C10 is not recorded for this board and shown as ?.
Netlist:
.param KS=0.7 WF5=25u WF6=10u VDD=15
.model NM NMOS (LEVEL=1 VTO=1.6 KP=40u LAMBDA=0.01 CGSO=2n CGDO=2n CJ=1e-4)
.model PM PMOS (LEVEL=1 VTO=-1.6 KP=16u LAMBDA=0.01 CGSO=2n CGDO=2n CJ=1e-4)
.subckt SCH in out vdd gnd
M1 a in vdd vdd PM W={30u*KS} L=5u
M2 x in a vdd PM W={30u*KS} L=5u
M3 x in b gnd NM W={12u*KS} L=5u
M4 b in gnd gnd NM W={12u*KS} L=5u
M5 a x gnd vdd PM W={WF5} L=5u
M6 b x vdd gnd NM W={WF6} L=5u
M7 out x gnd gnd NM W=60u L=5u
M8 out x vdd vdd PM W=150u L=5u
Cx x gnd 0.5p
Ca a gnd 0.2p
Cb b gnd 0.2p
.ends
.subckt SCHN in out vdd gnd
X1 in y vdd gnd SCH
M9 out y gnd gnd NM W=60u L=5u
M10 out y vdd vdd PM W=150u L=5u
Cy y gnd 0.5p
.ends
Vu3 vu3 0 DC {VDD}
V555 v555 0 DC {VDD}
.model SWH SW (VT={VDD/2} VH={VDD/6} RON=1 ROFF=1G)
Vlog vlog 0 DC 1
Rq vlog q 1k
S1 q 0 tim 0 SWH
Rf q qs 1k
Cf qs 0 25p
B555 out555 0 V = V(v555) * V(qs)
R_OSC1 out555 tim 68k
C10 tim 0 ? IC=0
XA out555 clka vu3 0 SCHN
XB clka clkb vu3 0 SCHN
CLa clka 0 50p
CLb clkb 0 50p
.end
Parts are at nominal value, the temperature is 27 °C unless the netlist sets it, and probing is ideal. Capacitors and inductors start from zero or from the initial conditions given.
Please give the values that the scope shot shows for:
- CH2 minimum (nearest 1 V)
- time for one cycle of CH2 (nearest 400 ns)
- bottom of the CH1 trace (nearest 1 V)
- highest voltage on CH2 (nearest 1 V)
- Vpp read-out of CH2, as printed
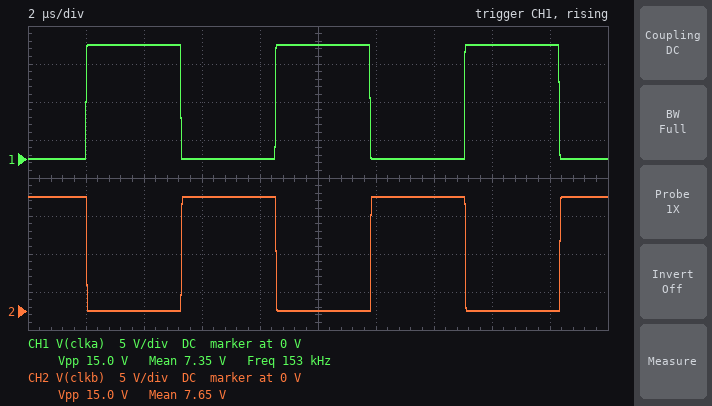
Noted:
0 V
6.4 µs
0 V
15 V
15.0 V
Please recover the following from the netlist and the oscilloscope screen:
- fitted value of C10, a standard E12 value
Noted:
68 pF
